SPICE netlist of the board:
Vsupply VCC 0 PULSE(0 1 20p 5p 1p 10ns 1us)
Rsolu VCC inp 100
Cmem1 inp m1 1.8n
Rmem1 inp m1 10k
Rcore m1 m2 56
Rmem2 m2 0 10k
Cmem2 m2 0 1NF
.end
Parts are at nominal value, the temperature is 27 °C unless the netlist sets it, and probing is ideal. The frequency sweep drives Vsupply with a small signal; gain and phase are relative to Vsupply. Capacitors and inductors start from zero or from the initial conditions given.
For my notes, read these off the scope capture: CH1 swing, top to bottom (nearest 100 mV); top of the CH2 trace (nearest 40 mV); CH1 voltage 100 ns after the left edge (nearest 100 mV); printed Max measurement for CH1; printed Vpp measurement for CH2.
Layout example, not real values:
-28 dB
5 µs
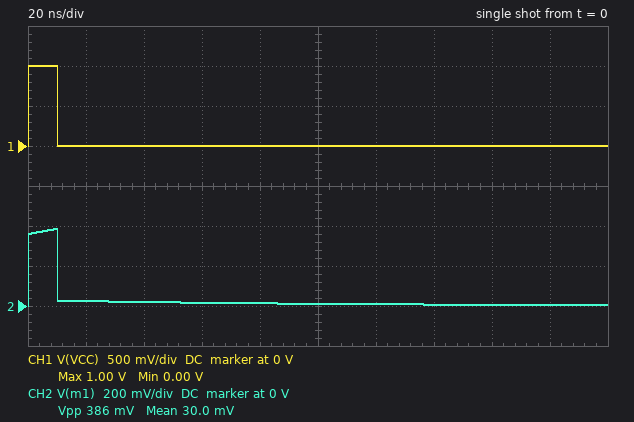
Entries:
1.0 V
400 mV
0 V
1.00 V
386 mV
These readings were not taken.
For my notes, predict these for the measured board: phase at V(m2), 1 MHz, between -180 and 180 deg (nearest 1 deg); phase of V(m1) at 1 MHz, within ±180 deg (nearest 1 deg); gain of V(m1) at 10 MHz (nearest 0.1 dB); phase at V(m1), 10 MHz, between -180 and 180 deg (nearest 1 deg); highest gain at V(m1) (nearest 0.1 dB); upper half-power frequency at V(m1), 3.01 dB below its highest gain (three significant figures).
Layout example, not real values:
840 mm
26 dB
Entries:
-32 deg
-13 deg
-8.7 dB
-7 deg
-3.9 dB
2.66 MHz
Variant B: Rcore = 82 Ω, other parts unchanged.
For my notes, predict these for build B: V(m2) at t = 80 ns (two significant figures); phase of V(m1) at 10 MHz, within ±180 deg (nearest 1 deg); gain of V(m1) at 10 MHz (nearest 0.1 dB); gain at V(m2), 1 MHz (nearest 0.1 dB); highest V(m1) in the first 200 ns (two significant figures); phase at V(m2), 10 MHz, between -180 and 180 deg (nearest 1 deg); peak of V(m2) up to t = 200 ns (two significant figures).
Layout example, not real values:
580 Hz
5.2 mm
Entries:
29 mV
-3 deg
-6.8 dB
-5.8 dB
470 mV
-82 deg
53 mV
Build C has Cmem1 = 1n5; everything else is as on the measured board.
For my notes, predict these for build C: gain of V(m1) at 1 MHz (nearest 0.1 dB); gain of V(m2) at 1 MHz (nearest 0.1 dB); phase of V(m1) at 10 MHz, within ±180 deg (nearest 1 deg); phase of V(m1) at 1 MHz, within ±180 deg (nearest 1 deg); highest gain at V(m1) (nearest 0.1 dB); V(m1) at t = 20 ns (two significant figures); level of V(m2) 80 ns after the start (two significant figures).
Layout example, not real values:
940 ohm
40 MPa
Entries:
-5.2 dB
-5.8 dB
-6 deg
-11 deg
-4.5 dB
22 mV
29 mV
